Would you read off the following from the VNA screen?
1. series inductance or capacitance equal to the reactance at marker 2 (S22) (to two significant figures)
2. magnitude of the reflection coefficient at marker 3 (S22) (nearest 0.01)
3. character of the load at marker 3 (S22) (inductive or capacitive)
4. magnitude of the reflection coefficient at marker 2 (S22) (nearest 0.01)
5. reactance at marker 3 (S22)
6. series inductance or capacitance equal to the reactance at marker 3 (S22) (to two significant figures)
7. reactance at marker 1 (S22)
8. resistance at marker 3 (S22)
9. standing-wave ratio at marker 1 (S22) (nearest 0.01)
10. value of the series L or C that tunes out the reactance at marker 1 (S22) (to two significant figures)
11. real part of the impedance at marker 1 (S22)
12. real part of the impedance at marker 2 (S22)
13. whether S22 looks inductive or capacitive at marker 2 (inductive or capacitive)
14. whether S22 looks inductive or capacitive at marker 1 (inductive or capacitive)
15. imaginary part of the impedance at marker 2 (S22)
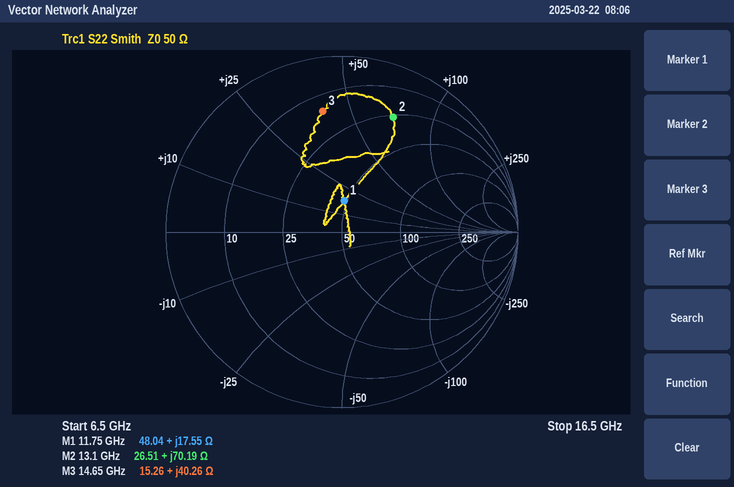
850 pH
0.69
inductive
0.71
+40.26 Ω
440 pH
+17.55 Ω
15.26 Ω
1.43
770 fF
48.04 Ω
26.51 Ω
inductive
inductive
+70.19 Ω
